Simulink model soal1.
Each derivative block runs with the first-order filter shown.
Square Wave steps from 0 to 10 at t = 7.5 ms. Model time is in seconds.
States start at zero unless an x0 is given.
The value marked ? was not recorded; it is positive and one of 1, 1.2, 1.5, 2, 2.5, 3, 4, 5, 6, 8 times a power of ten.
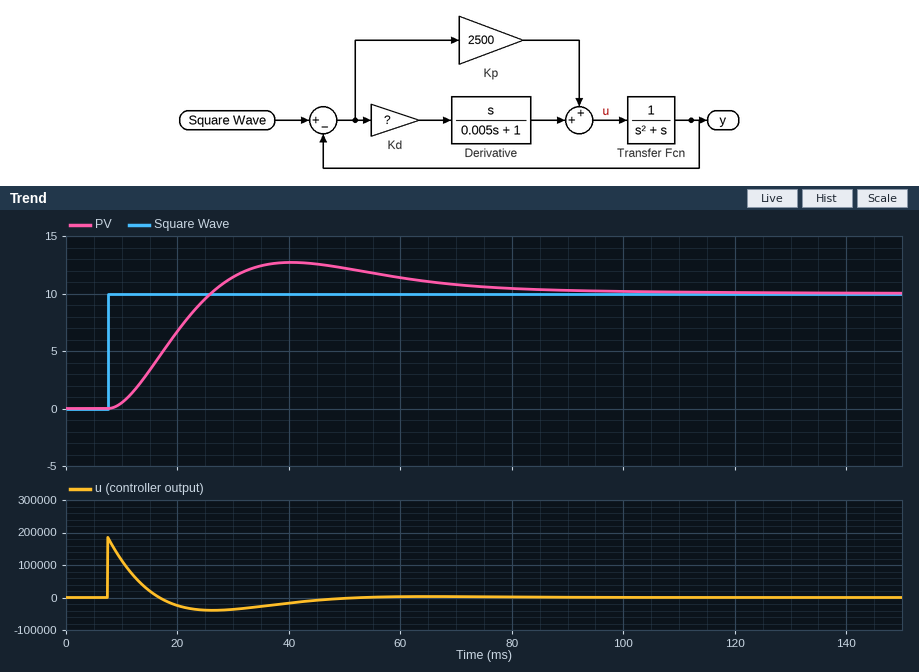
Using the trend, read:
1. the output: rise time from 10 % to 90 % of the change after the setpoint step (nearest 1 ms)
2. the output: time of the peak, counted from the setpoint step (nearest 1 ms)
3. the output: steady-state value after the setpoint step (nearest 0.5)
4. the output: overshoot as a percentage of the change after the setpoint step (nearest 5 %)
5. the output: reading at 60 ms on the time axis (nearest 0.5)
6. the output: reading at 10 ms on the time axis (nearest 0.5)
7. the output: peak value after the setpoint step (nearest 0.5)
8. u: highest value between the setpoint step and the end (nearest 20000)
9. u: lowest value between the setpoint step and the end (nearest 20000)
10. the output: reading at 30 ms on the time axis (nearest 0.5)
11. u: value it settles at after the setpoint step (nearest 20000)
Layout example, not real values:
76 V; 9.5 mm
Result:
13 ms; 33 ms; 10.0; 25 %; 11.5; 0.5; 12.5; 180000; -40000; 11.5; 0
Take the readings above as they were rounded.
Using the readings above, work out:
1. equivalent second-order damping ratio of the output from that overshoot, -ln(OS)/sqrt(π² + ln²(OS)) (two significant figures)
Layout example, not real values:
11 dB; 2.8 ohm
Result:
0.40
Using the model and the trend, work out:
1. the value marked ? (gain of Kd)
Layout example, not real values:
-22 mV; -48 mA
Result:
80
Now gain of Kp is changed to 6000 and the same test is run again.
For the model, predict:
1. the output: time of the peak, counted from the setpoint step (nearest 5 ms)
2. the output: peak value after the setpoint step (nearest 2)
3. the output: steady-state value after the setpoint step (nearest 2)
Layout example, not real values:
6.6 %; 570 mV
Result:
25 ms; 14; 10
